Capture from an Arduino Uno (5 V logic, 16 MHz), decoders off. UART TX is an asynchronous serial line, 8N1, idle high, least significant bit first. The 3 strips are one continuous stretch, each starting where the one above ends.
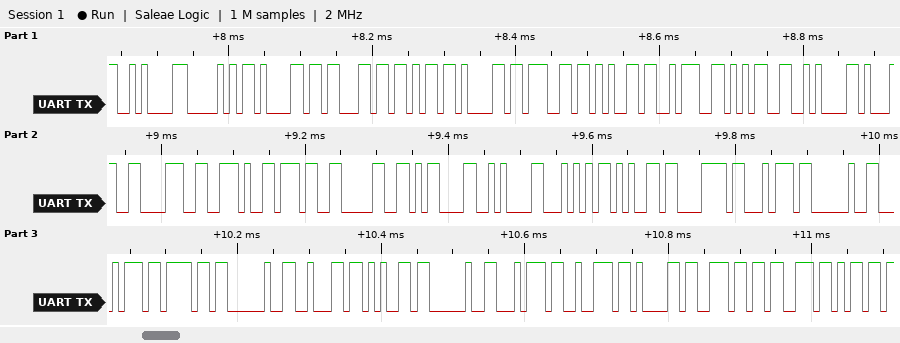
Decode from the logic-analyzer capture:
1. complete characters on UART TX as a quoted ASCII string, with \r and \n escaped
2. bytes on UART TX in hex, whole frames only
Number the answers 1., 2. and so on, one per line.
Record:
1. "\nPackage:5\n18.70\r\nText to be transm"
2. 0A 50 61 63 6B 61 67 65 3A 35 0A 31 38 2E 37 30 0D 0A 54 65 78 74 20 74 6F 20 62 65 20 74 72 61 6E 73 6D
